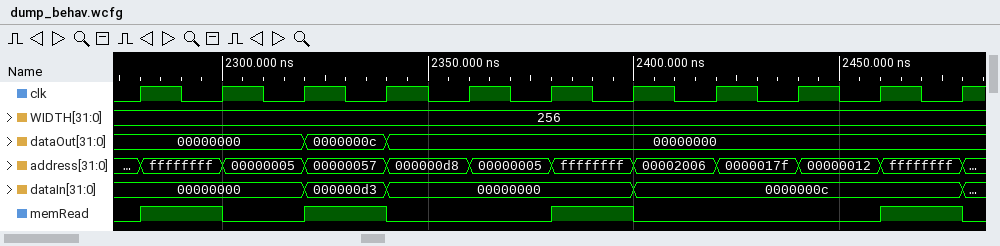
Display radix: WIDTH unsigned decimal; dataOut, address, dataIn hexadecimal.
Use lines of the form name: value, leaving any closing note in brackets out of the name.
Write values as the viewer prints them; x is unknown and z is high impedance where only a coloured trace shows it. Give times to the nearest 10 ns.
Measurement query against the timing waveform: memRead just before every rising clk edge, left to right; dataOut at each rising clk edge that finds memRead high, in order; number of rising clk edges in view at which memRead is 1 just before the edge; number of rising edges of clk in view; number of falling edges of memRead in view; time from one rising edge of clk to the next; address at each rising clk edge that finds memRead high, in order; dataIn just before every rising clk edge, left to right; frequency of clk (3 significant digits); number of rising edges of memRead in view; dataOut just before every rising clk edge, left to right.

memRead just before every rising clk edge, left to right: 0 1 0 1 0 0 1 0 0 0 1
dataOut at each rising clk edge that finds memRead high, in order: 00000000, 0000000c, 00000000, 00000000
number of rising clk edges in view at which memRead is 1 just before the edge: 4
number of rising edges of clk in view: 11
number of falling edges of memRead in view: 4
time from one rising edge of clk to the next: 20 ns
address at each rising clk edge that finds memRead high, in order: ffffffff, 00000057, ffffffff, ffffffff
dataIn just before every rising clk edge, left to right: 00000000, 00000000, 00000000, 000000d3, 00000000, 00000000, 00000000, 0000000c, 0000000c, 0000000c, 0000000c
frequency of clk: 50.0 MHz
number of rising edges of memRead in view: 4
dataOut just before every rising clk edge, left to right: 00000000, 00000000, 00000000, 0000000c, 00000000, 00000000, 00000000, 00000000, 00000000, 00000000, 00000000
